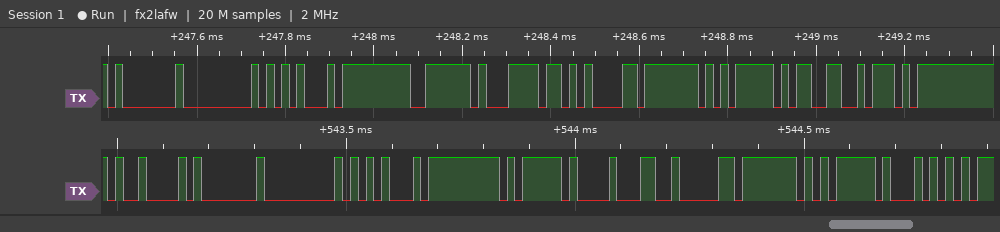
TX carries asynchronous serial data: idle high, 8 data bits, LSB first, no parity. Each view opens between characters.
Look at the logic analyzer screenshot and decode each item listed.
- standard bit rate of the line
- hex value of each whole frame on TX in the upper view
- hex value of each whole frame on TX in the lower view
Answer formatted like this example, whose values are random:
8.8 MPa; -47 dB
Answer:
57600 baud; 01, 00, 15, FF, 7E, BC, 85, 7F, 7D, 33, D7; 09, 01, 00, 15, FF, 7D, 88, 82, 7F, 7D, 54
